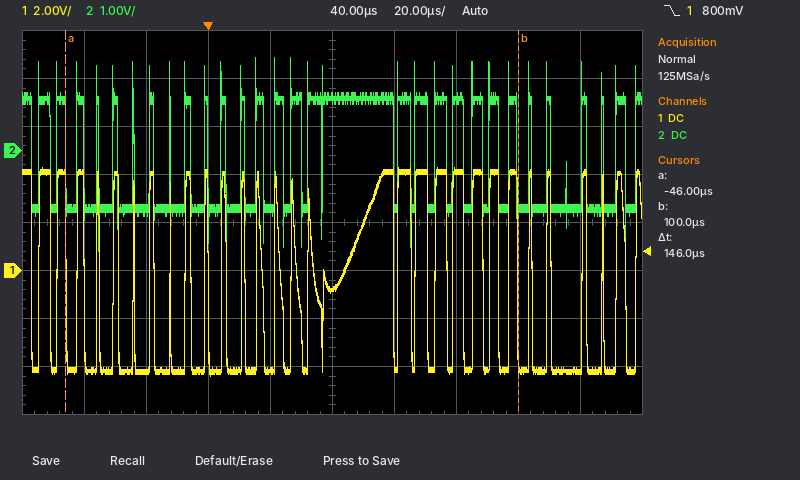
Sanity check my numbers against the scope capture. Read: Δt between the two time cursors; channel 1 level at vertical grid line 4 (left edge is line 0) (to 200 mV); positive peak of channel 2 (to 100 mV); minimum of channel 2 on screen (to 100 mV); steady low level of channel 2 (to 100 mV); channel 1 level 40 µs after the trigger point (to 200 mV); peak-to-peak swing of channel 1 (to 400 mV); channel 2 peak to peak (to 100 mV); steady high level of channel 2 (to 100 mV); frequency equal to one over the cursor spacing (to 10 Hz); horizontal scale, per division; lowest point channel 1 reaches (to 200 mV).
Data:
146 µs
-4.2 V
1.9 V
-2.1 V
-1.2 V
-800 mV
8.8 V
4.0 V
1.1 V
6.85 kHz
20 µs
-4.4 V
